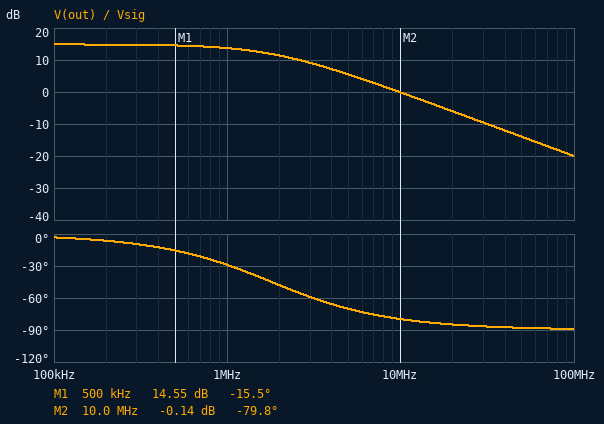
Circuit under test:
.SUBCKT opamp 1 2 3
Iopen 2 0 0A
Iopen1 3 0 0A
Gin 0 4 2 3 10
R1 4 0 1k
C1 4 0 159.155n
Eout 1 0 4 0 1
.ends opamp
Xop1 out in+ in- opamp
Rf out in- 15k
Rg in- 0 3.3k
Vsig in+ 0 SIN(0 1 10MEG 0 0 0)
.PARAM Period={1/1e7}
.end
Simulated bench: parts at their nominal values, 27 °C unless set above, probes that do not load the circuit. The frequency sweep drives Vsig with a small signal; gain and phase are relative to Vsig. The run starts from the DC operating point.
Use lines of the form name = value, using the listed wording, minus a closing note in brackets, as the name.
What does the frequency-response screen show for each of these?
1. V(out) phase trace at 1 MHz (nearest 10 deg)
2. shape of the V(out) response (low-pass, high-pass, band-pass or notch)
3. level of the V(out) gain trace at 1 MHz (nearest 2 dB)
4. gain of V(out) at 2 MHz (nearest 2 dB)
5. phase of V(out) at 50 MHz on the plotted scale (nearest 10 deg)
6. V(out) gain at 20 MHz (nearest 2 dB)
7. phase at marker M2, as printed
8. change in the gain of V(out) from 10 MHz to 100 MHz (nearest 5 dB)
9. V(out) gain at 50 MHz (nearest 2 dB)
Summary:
V(out) phase trace at 1 MHz = -30 deg
shape of the V(out) response = low-pass
level of the V(out) gain trace at 1 MHz = 14 dB
gain of V(out) at 2 MHz = 12 dB
phase of V(out) at 50 MHz on the plotted scale = -90 deg
V(out) gain at 20 MHz = -6 dB
phase at marker M2, as printed = -79.8 deg
change in the gain of V(out) from 10 MHz to 100 MHz = -20 dB
V(out) gain at 50 MHz = -14 dB
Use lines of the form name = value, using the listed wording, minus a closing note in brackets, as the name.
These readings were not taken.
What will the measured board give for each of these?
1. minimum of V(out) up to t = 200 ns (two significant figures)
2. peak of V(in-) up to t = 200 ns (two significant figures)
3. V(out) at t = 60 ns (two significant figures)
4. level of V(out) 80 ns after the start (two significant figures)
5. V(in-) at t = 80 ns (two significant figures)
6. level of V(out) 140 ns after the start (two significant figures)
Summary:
minimum of V(out) up to t = 200 ns = -880 mV
peak of V(in-) up to t = 200 ns = 280 mV
V(out) at t = 60 ns = 1.2 V
level of V(out) 80 ns after the start = -74 mV
V(in-) at t = 80 ns = -13 mV
level of V(out) 140 ns after the start = 1.1 V
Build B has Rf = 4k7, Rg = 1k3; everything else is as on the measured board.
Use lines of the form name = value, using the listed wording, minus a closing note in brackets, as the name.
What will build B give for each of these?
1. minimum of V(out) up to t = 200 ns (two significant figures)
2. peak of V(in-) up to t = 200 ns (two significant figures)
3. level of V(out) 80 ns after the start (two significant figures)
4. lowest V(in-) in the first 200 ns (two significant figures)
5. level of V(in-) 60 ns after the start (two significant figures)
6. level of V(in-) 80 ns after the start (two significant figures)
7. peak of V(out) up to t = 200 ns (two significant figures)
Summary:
minimum of V(out) up to t = 200 ns = -910 mV
peak of V(in-) up to t = 200 ns = 320 mV
level of V(out) 80 ns after the start = -170 mV
lowest V(in-) in the first 200 ns = -200 mV
level of V(in-) 60 ns after the start = 230 mV
level of V(in-) 80 ns after the start = -37 mV
peak of V(out) up to t = 200 ns = 1.5 V
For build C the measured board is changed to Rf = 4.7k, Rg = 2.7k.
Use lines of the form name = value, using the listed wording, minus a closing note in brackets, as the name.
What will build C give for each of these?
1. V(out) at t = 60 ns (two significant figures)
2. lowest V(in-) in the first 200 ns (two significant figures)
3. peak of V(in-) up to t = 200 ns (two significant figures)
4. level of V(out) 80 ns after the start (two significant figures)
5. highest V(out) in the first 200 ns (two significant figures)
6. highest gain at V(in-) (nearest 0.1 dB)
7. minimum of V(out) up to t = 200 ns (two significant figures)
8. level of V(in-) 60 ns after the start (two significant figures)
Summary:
V(out) at t = 60 ns = 750 mV
lowest V(in-) in the first 200 ns = -340 mV
peak of V(in-) up to t = 200 ns = 460 mV
level of V(out) 80 ns after the start = -440 mV
highest V(out) in the first 200 ns = 1.3 V
highest gain at V(in-) = 0 dB
minimum of V(out) up to t = 200 ns = -930 mV
level of V(in-) 60 ns after the start = 270 mV
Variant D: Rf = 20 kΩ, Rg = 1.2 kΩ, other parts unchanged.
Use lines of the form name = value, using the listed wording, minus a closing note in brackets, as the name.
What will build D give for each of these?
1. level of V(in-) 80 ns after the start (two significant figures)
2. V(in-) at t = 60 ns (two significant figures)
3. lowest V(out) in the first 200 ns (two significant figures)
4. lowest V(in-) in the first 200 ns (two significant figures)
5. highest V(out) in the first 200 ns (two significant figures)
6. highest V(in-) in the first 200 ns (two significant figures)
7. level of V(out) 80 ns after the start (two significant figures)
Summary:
level of V(in-) 80 ns after the start = 22 mV
V(in-) at t = 60 ns = 89 mV
lowest V(out) in the first 200 ns = -510 mV
lowest V(in-) in the first 200 ns = -29 mV
highest V(out) in the first 200 ns = 1.8 V
highest V(in-) in the first 200 ns = 100 mV
level of V(out) 80 ns after the start = 390 mV
